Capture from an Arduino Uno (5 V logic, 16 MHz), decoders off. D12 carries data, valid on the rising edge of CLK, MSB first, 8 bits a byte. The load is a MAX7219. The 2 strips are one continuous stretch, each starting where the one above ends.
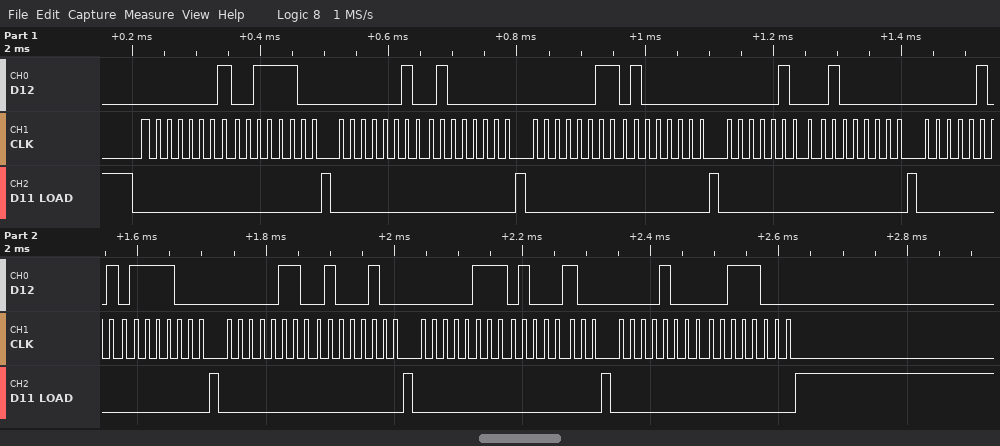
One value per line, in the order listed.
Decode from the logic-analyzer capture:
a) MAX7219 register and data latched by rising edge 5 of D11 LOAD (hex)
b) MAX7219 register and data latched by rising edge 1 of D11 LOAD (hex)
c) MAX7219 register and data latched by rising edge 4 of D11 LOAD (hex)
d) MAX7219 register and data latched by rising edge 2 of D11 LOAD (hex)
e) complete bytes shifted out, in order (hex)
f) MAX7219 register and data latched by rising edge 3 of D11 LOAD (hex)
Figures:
register 0x5, data 0x78
register 0x1, data 0x3C
register 0x4, data 0x40
register 0x2, data 0x40
0x01 0x3C 0x02 0x40 0x03 0x40 0x04 0x40 0x05 0x78 0x06 0x44 0x07 0x44 0x08 0x38
register 0x3, data 0x40
